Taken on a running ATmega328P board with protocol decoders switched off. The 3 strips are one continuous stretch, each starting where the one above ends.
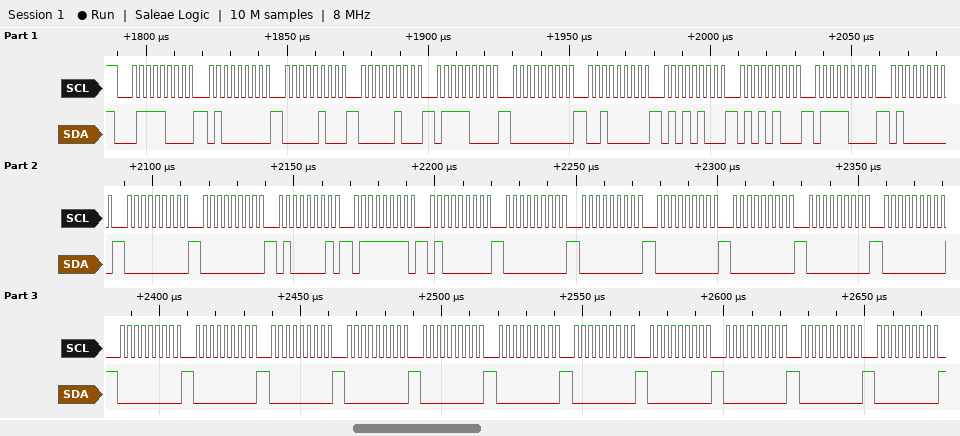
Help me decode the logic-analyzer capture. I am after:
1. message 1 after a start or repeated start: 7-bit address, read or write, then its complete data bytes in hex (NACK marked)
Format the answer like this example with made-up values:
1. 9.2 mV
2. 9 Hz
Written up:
1. 0x3C write: 40 04 04 78 00 20 54 54 78 40 00 00 41 7F 40 00 00 00 00 00 00 00 00 00 00 00 00 00 00 00 00 00
